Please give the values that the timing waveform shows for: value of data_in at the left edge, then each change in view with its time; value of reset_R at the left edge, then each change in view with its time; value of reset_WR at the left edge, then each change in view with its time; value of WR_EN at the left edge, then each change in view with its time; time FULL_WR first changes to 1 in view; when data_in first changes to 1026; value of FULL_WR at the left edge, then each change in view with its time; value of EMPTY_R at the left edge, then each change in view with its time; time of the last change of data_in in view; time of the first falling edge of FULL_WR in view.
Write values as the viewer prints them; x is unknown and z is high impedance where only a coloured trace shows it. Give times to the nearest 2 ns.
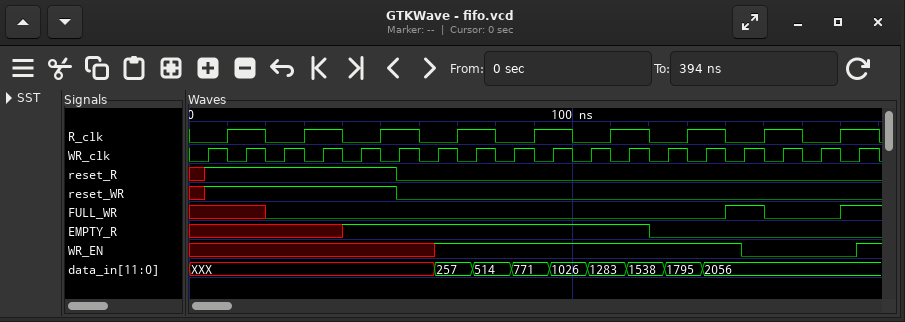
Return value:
XXX, 257 at 64 ns, 514 at 74 ns, 771 at 84 ns, 1026 at 94 ns, 1283 at 104 ns, 1538 at 114 ns, 1795 at 124 ns, 2056 at 134 ns
x, 1 at 4 ns, 0 at 54 ns
x, 1 at 4 ns, 0 at 54 ns
x, 1 at 64 ns, 0 at 144 ns, 1 at 174 ns
140 ns
94 ns
x, 0 at 20 ns, 1 at 140 ns, 0 at 150 ns, 1 at 170 ns
x, 1 at 40 ns, 0 at 120 ns
134 ns
150 ns
